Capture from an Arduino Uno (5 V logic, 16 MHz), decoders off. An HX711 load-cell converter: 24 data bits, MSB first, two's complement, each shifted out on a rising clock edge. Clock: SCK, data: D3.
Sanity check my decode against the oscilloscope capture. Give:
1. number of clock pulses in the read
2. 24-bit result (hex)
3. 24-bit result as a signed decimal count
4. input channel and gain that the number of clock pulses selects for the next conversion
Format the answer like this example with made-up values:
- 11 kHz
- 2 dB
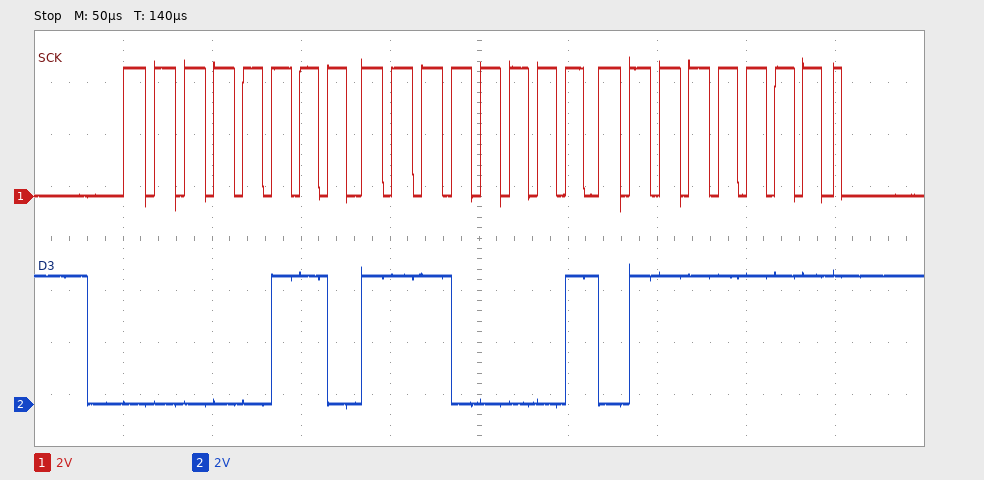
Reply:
- 25
- 0x06E17F
- 450943
- channel A, gain 128
